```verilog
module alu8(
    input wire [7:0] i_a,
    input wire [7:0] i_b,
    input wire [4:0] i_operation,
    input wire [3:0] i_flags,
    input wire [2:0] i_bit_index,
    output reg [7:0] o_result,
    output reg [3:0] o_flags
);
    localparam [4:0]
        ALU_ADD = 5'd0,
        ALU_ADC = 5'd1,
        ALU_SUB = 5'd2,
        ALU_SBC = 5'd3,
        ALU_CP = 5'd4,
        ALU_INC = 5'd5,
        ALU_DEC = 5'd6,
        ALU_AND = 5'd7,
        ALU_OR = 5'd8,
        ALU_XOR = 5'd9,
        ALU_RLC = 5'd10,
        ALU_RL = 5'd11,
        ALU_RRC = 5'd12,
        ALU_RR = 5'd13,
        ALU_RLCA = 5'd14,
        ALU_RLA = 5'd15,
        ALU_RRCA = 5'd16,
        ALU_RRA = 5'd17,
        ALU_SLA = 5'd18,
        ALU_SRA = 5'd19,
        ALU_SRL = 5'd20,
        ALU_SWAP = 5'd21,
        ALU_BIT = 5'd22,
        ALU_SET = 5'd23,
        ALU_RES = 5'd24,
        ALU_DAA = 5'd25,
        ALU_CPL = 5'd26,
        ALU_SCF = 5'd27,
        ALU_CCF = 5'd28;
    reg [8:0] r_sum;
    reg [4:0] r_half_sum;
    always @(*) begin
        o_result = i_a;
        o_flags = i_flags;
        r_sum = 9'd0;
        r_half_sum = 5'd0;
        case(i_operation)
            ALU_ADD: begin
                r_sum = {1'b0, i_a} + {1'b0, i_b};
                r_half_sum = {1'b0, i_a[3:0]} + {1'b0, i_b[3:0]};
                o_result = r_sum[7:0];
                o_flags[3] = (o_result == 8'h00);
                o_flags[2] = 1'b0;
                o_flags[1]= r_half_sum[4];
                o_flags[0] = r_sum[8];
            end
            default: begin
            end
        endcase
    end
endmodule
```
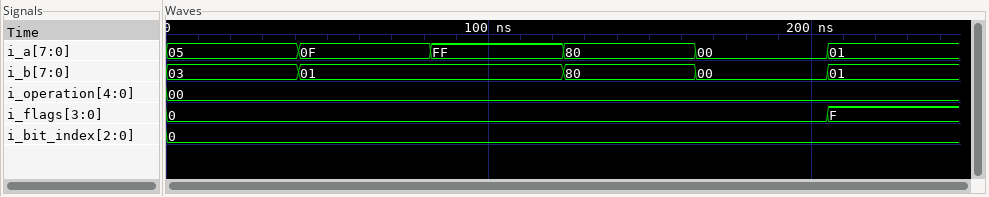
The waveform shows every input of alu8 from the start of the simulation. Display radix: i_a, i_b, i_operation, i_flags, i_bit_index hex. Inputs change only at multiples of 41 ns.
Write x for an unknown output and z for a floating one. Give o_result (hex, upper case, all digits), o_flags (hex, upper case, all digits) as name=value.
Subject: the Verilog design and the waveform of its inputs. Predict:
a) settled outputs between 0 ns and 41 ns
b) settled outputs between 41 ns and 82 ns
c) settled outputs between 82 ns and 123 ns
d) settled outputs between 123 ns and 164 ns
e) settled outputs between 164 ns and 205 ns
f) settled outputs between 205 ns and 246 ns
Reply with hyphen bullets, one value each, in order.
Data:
- o_result=08, o_flags=0
- o_result=10, o_flags=2
- o_result=00, o_flags=B
- o_result=00, o_flags=9
- o_result=00, o_flags=8
- o_result=02, o_flags=0
